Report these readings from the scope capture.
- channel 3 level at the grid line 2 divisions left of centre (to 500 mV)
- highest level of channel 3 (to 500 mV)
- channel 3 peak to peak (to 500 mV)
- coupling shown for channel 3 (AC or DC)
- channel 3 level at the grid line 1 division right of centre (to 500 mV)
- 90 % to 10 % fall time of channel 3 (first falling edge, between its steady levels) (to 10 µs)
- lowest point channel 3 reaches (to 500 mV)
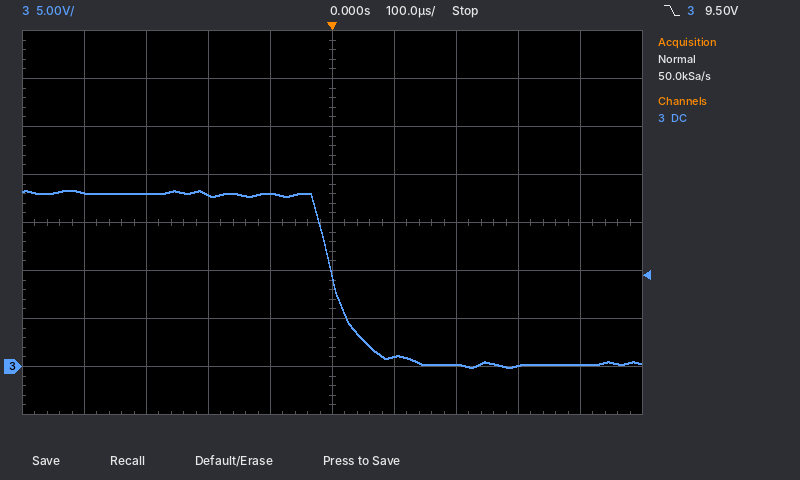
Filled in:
18.0 V
18.5 V
18.5 V
DC
1.0 V
90 µs
0.0 V
